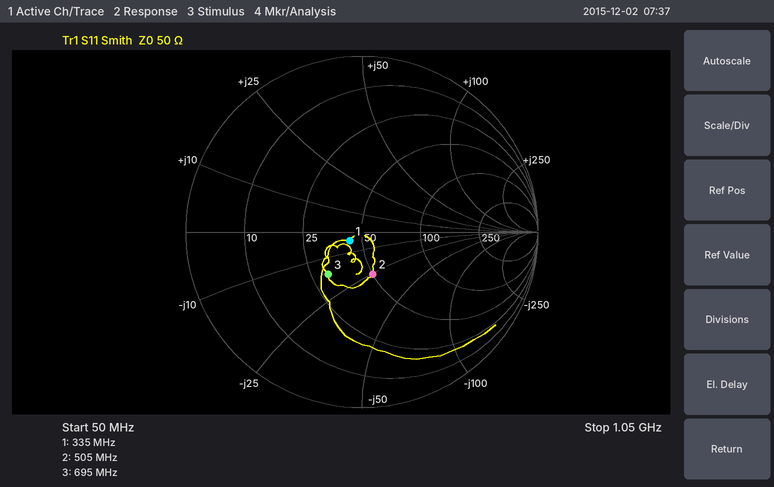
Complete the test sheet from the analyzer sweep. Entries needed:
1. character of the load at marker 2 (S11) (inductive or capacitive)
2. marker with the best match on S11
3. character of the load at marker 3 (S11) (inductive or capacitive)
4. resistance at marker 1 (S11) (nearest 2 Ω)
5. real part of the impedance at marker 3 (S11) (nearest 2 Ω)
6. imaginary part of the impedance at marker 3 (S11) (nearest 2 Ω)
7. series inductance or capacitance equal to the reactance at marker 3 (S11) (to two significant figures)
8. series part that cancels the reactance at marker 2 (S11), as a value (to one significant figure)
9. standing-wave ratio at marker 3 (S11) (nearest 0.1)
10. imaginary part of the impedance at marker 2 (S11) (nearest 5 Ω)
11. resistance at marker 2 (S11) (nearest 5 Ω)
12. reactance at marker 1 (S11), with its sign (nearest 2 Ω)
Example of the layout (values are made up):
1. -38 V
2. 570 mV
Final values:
1. capacitive
2. marker 1
3. capacitive
4. 44 Ω
5. 30 Ω
6. -16 Ω
7. 14 pF
8. 8 nH
9. 1.9
10. -25 Ω
11. 50 Ω
12. -4 Ω
